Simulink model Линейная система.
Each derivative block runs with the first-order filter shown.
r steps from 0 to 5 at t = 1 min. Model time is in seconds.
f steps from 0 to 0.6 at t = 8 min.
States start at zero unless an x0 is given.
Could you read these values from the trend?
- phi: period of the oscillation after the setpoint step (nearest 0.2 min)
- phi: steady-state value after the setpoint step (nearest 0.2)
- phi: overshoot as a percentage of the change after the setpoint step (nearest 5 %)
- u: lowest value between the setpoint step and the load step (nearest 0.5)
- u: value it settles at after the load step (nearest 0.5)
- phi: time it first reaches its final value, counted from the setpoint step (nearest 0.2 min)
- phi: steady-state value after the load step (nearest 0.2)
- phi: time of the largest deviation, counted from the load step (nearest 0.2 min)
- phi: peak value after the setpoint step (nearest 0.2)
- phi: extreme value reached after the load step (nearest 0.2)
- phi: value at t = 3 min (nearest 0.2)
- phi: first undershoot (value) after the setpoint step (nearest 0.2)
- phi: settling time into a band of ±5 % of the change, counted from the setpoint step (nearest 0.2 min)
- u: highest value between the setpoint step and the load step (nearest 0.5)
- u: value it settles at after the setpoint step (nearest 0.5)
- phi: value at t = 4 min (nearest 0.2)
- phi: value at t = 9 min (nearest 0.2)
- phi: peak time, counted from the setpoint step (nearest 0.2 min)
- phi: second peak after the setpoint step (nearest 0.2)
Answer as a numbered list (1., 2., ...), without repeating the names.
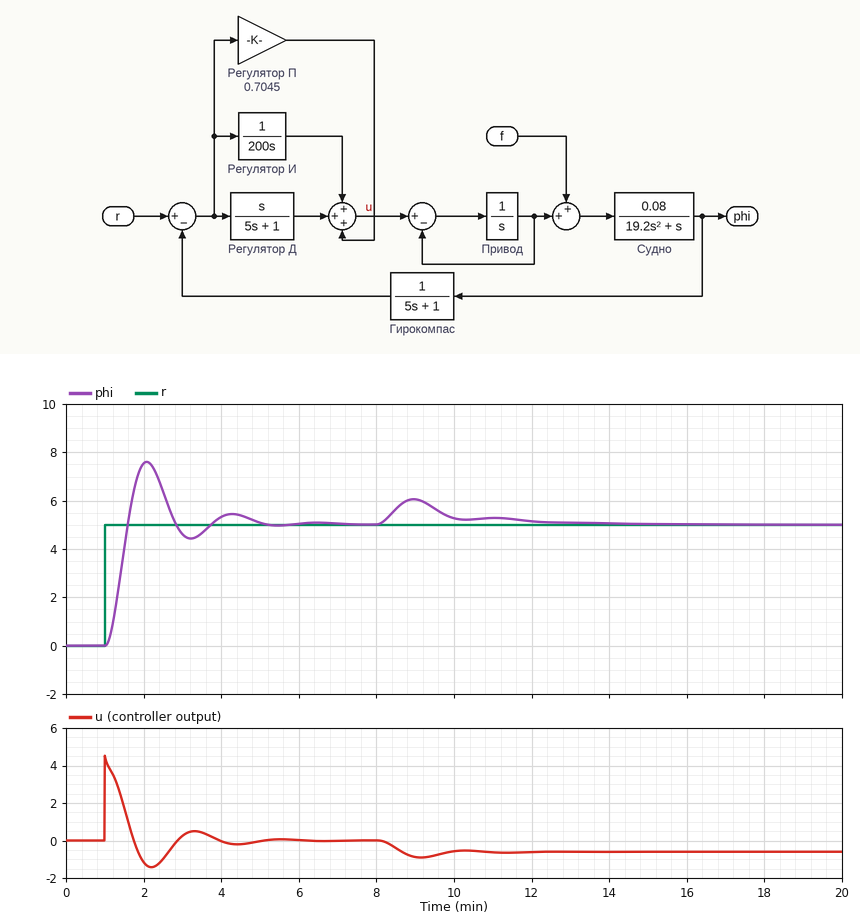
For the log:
1. 2.2 min
2. 5.0
3. 50 %
4. -1.5
5. -0.5
6. 0.6 min
7. 5.0
8. 1.0 min
9. 7.6
10. 6.0
11. 4.6
12. 4.4
13. 3.8 min
14. 4.5
15. 0.0
16. 5.4
17. 6.0
18. 1.0 min
19. 5.4
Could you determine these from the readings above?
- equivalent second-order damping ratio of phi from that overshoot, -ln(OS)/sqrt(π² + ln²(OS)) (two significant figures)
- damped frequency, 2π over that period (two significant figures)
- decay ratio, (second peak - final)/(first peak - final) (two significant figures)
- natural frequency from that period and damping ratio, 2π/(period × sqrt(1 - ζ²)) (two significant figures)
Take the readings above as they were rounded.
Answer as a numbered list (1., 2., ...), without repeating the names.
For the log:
1. 0.22
2. 2.9 rad/min
3. 0.15
4. 2.9 rad/min
